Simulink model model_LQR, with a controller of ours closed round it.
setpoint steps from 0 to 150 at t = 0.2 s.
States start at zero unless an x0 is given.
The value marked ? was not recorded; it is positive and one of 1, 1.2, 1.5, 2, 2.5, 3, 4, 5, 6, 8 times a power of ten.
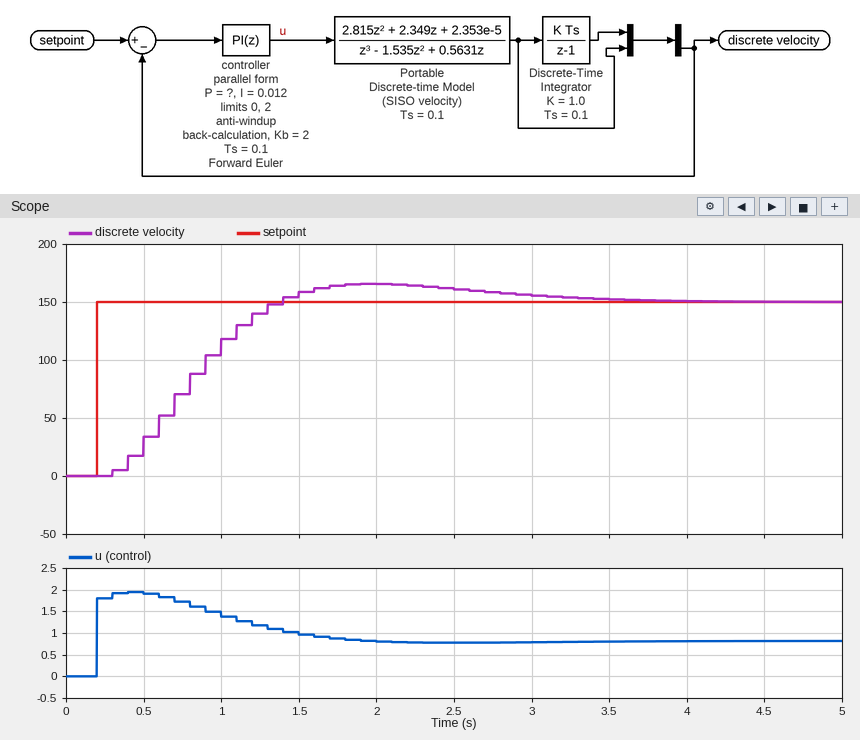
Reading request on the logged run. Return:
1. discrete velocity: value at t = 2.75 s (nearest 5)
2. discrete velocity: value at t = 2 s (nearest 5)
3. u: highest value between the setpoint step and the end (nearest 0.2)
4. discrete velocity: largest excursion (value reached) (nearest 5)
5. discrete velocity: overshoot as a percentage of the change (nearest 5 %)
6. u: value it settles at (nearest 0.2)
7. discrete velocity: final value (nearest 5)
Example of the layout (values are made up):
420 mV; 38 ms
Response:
160; 165; 2.0; 165; 10 %; 0.8; 150
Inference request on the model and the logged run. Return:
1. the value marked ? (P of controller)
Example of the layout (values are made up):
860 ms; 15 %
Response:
0.012
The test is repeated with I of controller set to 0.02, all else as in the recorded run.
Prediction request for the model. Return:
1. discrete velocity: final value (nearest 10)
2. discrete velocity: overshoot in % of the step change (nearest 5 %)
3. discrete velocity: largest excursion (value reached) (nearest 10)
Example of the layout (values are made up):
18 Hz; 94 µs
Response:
150; 25 %; 190
